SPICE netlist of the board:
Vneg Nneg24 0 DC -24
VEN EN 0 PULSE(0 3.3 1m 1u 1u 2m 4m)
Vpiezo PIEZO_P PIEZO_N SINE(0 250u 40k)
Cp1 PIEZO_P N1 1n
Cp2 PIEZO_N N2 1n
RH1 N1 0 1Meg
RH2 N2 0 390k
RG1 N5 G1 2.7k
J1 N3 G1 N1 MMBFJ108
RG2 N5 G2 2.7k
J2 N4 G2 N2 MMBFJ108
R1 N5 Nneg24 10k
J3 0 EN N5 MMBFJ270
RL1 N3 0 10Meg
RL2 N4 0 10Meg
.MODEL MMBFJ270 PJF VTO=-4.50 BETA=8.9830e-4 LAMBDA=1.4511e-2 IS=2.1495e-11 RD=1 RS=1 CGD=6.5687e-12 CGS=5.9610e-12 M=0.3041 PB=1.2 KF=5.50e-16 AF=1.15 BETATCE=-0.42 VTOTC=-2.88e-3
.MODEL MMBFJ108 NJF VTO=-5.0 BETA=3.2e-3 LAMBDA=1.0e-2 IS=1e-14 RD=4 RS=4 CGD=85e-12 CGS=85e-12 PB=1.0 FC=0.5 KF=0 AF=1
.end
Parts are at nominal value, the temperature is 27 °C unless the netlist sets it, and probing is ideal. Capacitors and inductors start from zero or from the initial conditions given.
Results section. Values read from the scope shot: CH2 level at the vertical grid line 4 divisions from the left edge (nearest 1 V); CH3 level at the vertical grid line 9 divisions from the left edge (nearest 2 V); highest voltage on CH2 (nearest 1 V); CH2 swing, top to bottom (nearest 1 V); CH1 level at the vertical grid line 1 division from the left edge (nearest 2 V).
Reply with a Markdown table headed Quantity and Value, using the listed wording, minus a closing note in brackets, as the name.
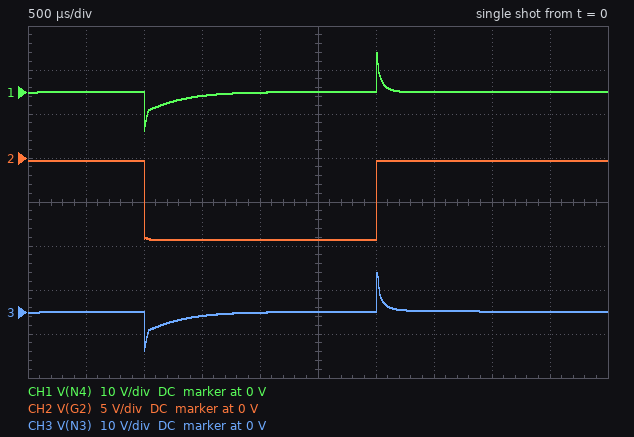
| Quantity | Value |
|---|---|
| CH2 level at the vertical grid line 4 divisions from the left edge | -9 V |
| CH3 level at the vertical grid line 9 divisions from the left edge | 0 V |
| highest voltage on CH2 | 0 V |
| CH2 swing, top to bottom | 9 V |
| CH1 level at the vertical grid line 1 division from the left edge | 0 V |
